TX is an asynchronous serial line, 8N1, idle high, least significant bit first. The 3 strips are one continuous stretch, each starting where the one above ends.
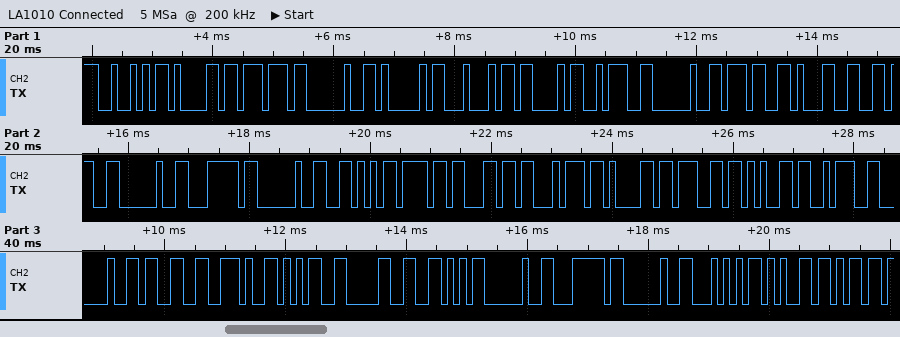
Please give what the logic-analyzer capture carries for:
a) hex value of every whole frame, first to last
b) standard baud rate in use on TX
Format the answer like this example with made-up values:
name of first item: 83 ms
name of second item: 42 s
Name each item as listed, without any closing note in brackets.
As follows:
hex value of every whole frame, first to last: 52 61 77 20 41 44 43 3A 20 37 31 36 20 7C 20 56 6F 6C 74 61 67 65 3A 20 33 2E 35 30 56 20 7C 20 54 65 6D
standard baud rate in use on TX: 9600 baud
